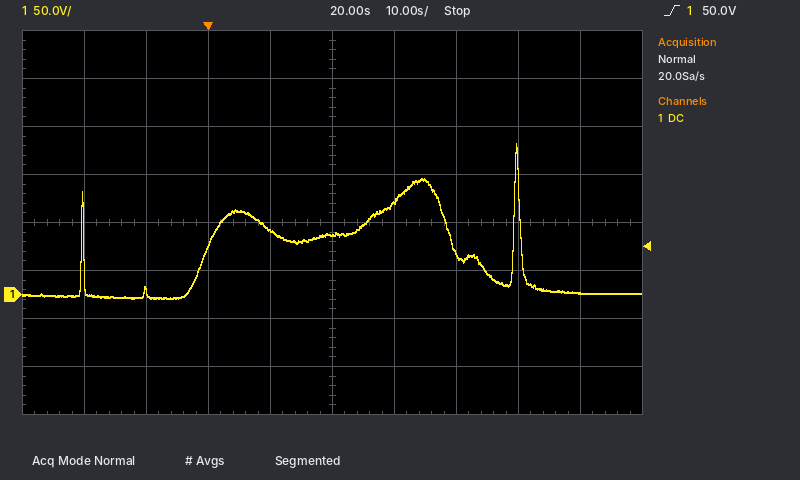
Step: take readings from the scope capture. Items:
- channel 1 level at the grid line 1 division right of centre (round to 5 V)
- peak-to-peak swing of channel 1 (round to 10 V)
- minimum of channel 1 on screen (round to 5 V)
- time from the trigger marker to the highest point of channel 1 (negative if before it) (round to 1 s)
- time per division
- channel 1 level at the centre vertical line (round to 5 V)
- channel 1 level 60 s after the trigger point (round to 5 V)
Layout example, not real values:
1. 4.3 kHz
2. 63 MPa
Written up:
1. 95 V
2. 160 V
3. -5 V
4. +50 s
5. 10 s
6. 60 V
7. 0 V
